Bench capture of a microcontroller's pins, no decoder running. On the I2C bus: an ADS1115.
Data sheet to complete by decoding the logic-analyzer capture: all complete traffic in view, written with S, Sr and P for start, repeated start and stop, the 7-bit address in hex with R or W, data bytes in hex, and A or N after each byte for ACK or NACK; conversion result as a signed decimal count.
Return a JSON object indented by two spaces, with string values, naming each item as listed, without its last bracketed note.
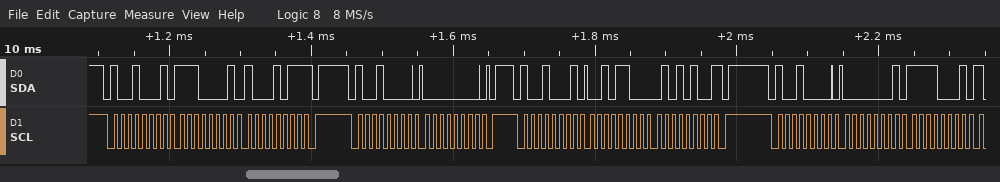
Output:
{
  "all complete traffic in view, written with S, Sr and P for start, repeated start and stop, the 7-bit address in hex with R or W, data bytes in hex, and A or N after each byte for ACK or NACK": "S 48R A E1 A 8B N P S 48W A 00 A P S 48R A 2C A 54 N P S 48W A 01 A F1 A",
  "conversion result as a signed decimal count": "11348"
}
